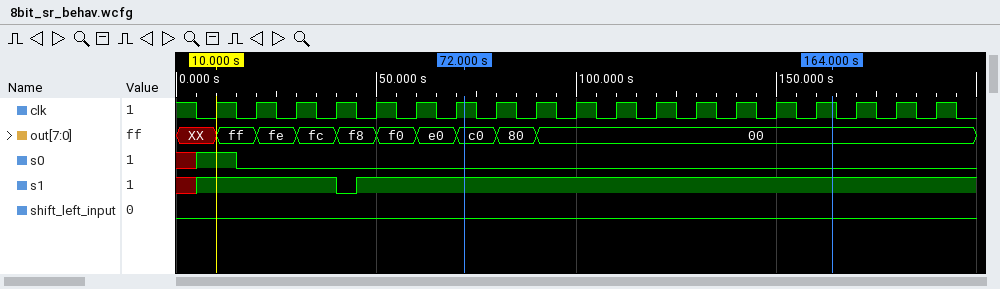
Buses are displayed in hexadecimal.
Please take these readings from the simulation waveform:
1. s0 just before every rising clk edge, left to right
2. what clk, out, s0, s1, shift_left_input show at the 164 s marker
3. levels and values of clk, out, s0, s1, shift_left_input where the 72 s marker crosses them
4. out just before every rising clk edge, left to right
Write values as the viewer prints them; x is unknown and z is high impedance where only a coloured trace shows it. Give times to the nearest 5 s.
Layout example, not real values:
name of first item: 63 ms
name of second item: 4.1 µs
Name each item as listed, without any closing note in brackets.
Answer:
s0 just before every rising clk edge, left to right: 1 0 0 0 0 0 0 0 0 0 0 0 0 0 0 0 0 0 0
what clk, out, s0, s1, shift_left_input show at the 164 s marker: clk=1, out=00, s0=0, s1=1, shift_left_input=0
levels and values of clk, out, s0, s1, shift_left_input where the 72 s marker crosses them: clk=1, out=c0, s0=0, s1=1, shift_left_input=0
out just before every rising clk edge, left to right: XX, ff, fe, fc, f8, f0, e0, c0, 80, 00, 00, 00, 00, 00, 00, 00, 00, 00, 00
